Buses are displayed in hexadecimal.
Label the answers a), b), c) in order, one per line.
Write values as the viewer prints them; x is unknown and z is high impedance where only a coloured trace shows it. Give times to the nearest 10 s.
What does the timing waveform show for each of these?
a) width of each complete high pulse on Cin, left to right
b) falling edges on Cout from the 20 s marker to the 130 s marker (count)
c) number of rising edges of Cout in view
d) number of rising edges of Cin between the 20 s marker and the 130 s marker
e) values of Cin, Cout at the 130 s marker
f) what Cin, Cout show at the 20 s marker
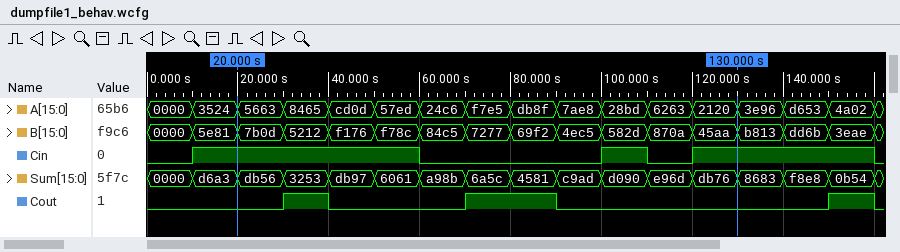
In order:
a) 50 s, 10 s, 40 s
b) 2
c) 3
d) 2
e) Cin=1, Cout=0
f) Cin=1, Cout=0
